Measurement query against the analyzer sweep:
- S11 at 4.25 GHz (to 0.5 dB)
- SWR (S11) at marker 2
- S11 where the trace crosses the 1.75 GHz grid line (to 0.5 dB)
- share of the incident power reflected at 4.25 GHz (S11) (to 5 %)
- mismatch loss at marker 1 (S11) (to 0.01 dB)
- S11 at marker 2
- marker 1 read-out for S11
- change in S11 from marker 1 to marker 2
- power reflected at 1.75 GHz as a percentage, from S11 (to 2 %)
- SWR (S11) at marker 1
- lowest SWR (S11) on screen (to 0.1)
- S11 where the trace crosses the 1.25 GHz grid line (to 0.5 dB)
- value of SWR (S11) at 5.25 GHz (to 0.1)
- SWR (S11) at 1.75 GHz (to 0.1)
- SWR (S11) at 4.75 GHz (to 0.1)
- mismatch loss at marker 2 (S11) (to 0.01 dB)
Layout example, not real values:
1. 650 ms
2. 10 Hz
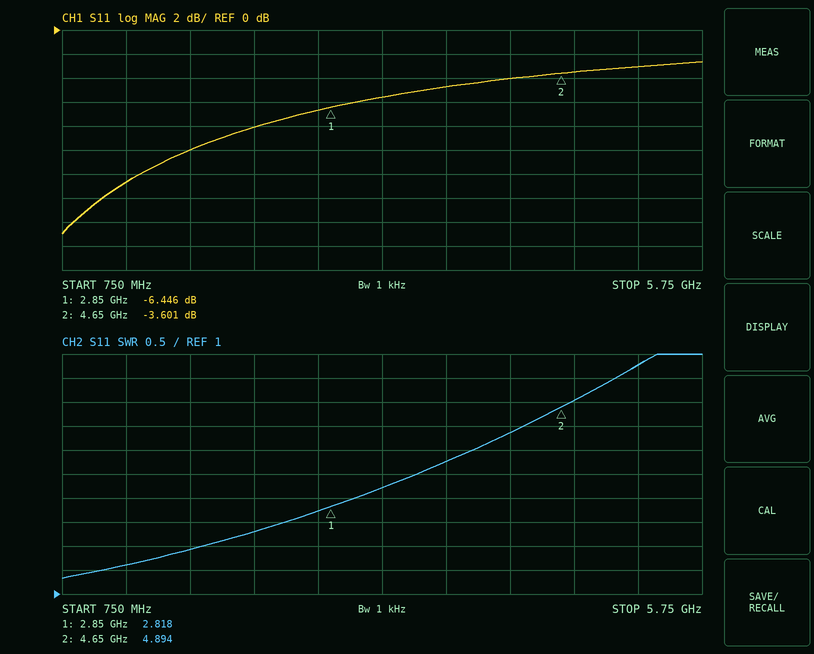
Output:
1. -4.0 dB
2. 4.894
3. -10.0 dB
4. 40 %
5. 1.12 dB
6. -3.601 dB
7. -6.446 dB
8. 2.845 dB
9. 10 %
10. 2.818
11. 1.3
12. -12.5 dB
13. 5.8
14. 1.9
15. 5.0
16. 2.49 dB
